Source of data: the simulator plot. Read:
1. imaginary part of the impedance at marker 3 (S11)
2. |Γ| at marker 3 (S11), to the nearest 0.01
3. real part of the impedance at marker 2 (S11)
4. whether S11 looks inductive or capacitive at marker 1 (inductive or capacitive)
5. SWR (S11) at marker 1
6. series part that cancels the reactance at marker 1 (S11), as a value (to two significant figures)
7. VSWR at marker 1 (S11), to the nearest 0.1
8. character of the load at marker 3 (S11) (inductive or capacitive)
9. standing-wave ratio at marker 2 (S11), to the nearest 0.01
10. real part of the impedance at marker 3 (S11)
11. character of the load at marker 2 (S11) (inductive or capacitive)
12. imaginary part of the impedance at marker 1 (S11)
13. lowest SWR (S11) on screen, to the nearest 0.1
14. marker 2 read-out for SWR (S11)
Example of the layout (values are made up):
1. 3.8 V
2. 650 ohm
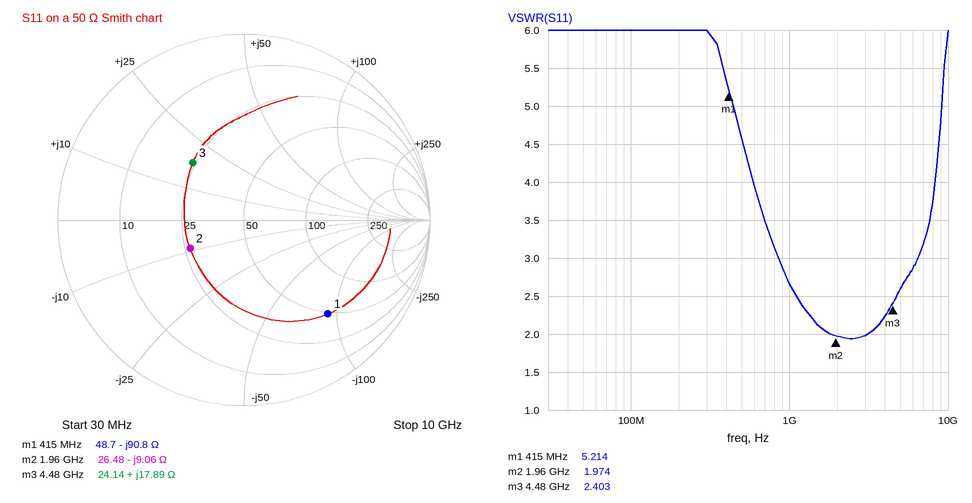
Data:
1. +17.89 Ω
2. 0.41
3. 26.48 Ω
4. capacitive
5. 5.214
6. 35 nH
7. 5.2
8. inductive
9. 1.97
10. 24.14 Ω
11. capacitive
12. -90.8 Ω
13. 1.9
14. 1.974
